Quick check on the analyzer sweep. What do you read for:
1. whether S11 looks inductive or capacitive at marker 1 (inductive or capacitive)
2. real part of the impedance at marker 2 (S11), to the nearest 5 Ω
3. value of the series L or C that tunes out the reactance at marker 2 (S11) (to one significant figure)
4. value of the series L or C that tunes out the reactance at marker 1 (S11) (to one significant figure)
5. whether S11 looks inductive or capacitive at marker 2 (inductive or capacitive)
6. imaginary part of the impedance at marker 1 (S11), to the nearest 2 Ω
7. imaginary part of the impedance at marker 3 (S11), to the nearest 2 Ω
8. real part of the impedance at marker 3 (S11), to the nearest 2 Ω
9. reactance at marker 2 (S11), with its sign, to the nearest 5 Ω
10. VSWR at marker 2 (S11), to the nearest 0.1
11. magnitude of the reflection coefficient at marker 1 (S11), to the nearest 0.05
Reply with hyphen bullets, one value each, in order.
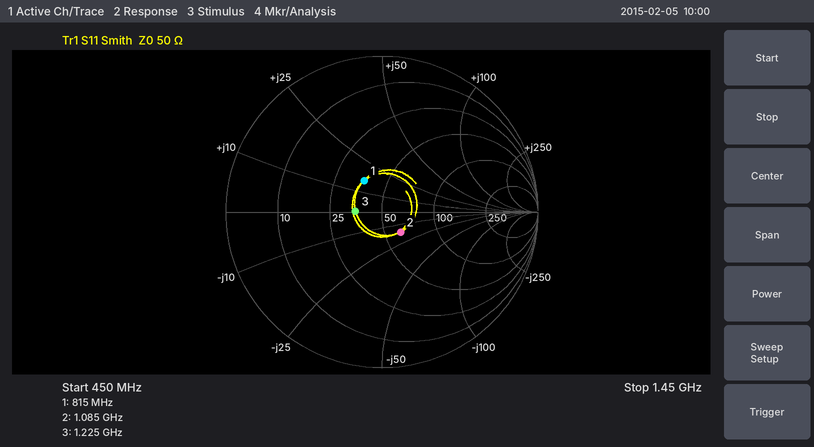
- inductive
- 60 Ω
- 2 nH
- 10 pF
- capacitive
- +16 Ω
- 0 Ω
- 36 Ω
- -15 Ω
- 1.4
- 0.25
